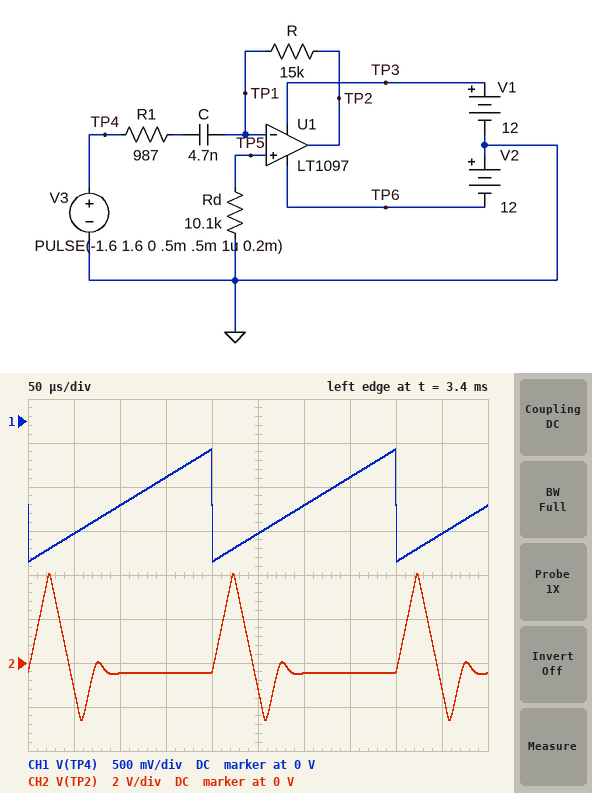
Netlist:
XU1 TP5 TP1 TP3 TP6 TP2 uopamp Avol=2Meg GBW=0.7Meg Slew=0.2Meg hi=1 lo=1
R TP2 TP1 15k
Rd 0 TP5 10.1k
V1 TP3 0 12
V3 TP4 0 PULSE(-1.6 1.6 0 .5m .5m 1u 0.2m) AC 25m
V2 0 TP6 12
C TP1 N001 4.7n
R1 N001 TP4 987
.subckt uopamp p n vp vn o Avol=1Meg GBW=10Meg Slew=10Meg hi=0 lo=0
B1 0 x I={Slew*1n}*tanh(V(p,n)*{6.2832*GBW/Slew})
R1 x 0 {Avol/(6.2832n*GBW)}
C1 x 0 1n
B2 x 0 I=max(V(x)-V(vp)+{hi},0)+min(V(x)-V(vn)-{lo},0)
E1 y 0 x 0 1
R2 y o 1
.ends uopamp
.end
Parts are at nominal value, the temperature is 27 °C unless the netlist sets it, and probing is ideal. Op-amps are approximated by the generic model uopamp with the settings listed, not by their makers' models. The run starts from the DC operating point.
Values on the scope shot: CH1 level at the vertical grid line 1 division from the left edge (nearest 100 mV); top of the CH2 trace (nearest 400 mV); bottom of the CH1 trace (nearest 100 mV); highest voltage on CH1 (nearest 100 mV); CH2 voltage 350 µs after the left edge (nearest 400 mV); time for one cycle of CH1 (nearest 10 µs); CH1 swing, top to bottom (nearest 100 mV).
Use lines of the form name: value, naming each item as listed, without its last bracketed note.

CH1 level at the vertical grid line 1 division from the left edge: -1.3 V
top of the CH2 trace: 4.0 V
bottom of the CH1 trace: -1.6 V
highest voltage on CH1: -300 mV
CH2 voltage 350 µs after the left edge: -400 mV
time for one cycle of CH1: 200 µs
CH1 swing, top to bottom: 1.3 V
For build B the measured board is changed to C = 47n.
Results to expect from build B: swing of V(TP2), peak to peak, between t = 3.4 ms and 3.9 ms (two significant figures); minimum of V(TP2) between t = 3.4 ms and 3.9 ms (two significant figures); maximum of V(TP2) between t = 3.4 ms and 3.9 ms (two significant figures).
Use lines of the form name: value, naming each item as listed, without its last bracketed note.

swing of V(TP2), peak to peak, between t = 3.4 ms and 3.9 ms: 11 V
minimum of V(TP2) between t = 3.4 ms and 3.9 ms: -4.1 V
maximum of V(TP2) between t = 3.4 ms and 3.9 ms: 7.0 V
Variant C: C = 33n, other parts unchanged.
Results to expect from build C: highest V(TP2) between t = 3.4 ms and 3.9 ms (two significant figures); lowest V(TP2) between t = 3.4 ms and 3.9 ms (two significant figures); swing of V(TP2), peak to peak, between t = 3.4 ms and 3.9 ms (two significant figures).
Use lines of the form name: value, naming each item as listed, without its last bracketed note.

highest V(TP2) between t = 3.4 ms and 3.9 ms: 7.0 V
lowest V(TP2) between t = 3.4 ms and 3.9 ms: -3.1 V
swing of V(TP2), peak to peak, between t = 3.4 ms and 3.9 ms: 10 V
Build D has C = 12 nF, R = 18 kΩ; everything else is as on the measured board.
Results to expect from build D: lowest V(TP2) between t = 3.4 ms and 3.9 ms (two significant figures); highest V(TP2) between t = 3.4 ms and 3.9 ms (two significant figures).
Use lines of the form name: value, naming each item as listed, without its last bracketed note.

lowest V(TP2) between t = 3.4 ms and 3.9 ms: -4.1 V
highest V(TP2) between t = 3.4 ms and 3.9 ms: 6.4 V
